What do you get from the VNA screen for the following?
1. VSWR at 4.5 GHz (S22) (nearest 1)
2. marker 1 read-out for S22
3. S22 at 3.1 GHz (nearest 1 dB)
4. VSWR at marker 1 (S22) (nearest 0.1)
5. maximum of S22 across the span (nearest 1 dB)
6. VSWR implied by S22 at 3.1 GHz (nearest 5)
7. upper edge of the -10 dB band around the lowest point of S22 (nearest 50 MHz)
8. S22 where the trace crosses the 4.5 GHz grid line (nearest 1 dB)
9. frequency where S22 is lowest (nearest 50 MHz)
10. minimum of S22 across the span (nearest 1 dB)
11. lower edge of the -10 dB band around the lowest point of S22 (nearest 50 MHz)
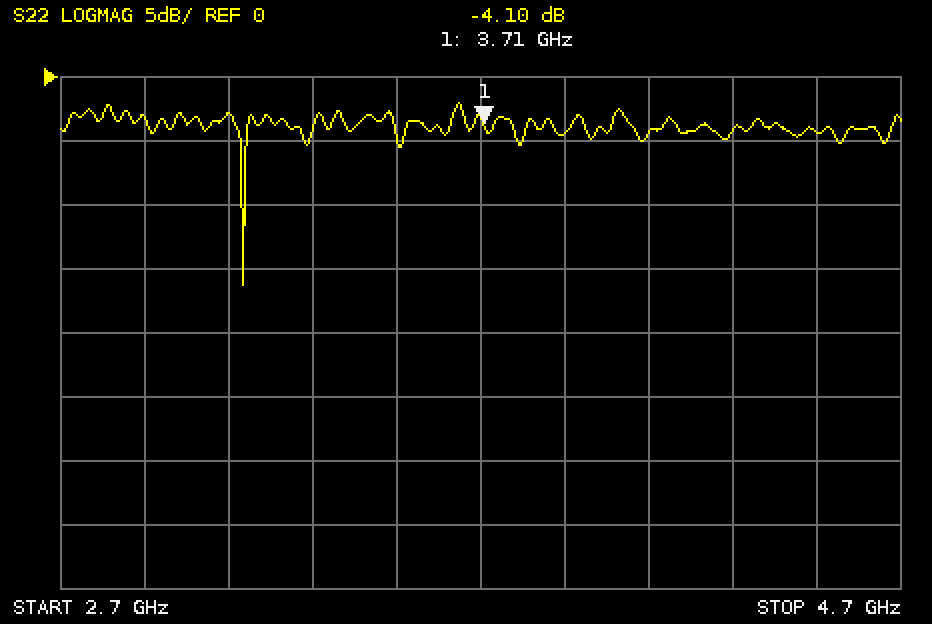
4
-4.10 dB
-3 dB
4.3
-2 dB
5
3.15 GHz
-4 dB
3.15 GHz
-16 dB
3.15 GHz
